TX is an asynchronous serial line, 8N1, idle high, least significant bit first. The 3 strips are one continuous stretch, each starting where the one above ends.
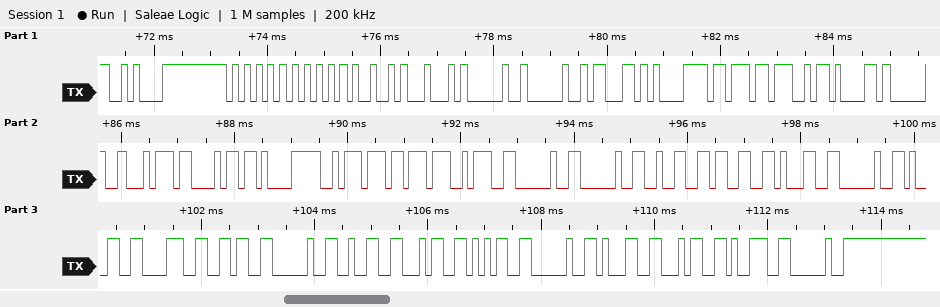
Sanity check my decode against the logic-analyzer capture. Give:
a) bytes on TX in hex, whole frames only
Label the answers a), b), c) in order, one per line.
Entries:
a) 0A 55 55 49 44 20 20 63 E1 BB A7 61 20 74 68 E1 BA BB 3A 20 20 32 33 31 20 31 38 36 20 32 34 35 20 31 34 39 20
